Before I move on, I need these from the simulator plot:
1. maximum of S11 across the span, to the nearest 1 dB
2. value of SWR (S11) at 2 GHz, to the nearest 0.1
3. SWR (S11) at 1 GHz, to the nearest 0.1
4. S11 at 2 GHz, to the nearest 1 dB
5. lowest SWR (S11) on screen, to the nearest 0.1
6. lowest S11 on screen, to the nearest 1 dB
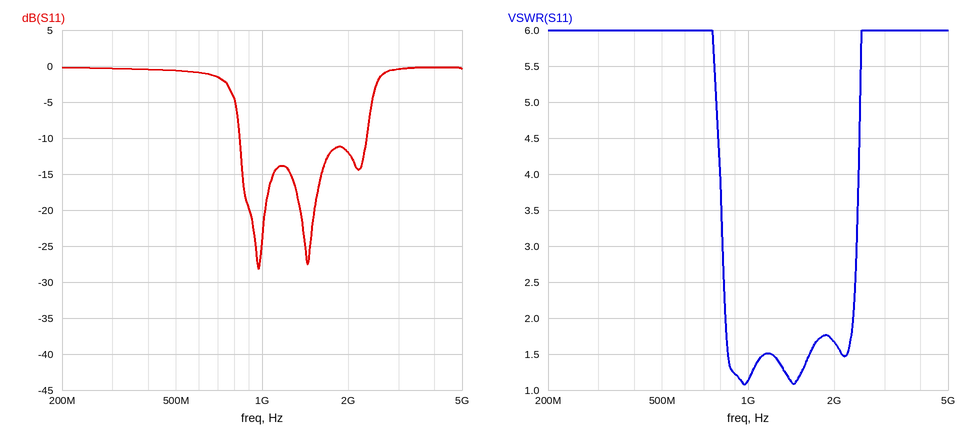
0 dB
1.7
1.1
-12 dB
1.1
-28 dB
